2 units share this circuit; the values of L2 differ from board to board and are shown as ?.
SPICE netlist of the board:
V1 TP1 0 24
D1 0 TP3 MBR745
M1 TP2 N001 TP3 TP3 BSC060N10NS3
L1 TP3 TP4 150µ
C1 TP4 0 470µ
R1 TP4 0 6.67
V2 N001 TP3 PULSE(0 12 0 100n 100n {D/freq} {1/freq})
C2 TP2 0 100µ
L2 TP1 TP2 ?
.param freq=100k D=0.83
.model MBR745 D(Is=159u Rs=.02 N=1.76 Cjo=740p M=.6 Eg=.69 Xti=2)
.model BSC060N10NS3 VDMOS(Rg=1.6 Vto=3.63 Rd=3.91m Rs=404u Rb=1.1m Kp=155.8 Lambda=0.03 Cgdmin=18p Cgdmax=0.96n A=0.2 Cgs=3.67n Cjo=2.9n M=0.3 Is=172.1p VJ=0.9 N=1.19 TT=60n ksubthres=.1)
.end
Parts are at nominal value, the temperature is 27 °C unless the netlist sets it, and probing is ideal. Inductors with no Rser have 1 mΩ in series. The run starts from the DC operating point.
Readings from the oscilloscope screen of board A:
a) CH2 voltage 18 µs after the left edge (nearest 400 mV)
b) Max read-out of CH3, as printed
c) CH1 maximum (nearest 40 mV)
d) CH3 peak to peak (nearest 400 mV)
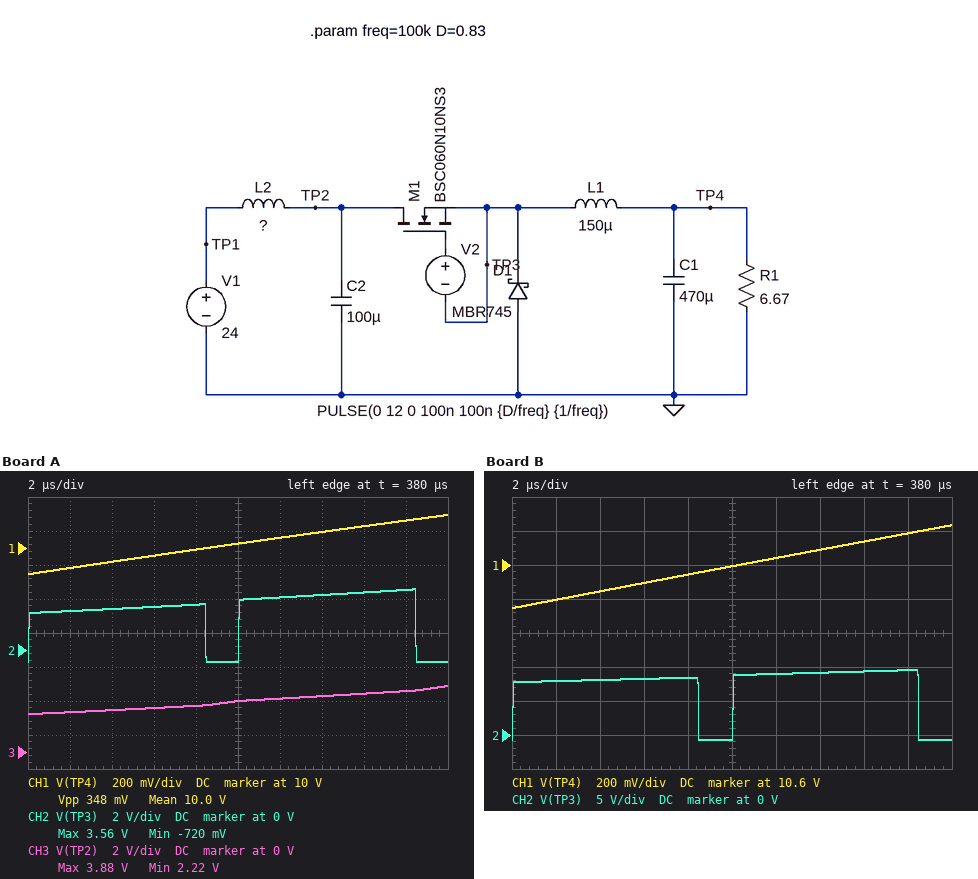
3.6 V
3.88 V
10.20 V
1.6 V
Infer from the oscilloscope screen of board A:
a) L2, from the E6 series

330 µH
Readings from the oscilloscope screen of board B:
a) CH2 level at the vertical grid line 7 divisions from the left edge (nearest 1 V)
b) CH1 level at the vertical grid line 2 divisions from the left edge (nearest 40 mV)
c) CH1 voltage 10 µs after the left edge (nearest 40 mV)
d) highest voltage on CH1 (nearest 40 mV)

9 V
10.44 V
10.60 V
10.84 V
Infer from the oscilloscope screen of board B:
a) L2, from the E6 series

220 µH
